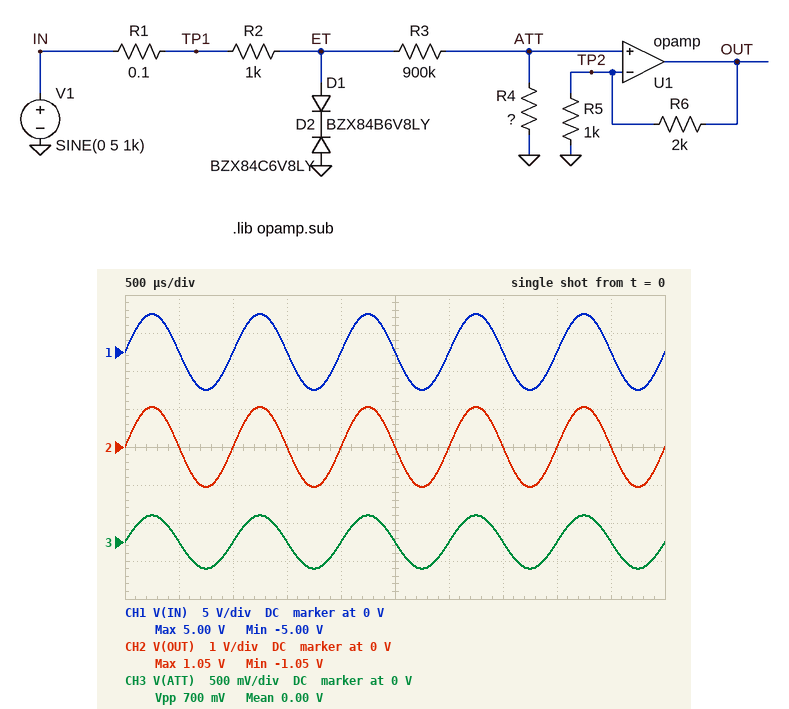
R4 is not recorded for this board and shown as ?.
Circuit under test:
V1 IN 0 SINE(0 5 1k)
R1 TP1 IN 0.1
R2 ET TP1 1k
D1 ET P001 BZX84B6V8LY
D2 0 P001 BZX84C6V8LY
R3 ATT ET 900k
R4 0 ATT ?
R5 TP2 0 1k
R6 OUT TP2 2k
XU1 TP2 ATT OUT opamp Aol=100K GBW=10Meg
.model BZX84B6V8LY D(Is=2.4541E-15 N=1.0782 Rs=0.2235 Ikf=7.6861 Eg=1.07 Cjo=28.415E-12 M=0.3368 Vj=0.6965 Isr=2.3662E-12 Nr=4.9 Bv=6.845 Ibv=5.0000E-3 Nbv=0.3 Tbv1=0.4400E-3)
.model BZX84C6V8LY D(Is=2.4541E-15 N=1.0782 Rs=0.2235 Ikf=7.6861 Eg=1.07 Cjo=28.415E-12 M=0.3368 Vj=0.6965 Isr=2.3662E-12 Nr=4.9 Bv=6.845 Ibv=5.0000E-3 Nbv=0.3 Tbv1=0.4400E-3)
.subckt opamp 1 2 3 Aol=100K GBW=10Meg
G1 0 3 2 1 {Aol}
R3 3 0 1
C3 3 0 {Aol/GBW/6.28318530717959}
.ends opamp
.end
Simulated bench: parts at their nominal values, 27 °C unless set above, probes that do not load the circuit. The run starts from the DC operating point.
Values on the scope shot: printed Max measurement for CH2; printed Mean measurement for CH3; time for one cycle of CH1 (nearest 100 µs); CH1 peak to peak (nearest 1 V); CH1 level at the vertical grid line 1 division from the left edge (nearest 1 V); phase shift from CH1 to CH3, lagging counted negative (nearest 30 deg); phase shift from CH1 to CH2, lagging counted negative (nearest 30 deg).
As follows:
1.05 V
0.00 V
1.0 ms
10 V
0 V
0 deg
0 deg
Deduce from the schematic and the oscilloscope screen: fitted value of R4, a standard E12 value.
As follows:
68 kΩ
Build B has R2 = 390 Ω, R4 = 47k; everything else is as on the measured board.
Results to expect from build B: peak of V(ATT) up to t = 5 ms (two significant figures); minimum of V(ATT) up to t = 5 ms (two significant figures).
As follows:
250 mV
-250 mV
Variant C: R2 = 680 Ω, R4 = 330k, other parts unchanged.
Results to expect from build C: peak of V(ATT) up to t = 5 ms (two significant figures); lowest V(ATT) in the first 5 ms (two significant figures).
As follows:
1.3 V
-1.3 V
